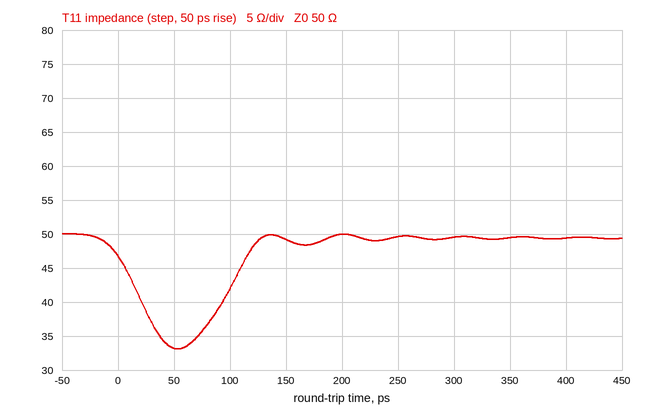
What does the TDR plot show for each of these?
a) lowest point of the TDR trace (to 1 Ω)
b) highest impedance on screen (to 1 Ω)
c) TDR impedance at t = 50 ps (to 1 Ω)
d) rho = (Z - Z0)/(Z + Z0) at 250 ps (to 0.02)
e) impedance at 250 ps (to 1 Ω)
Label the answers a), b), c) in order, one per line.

a) 33 Ω
b) 50 Ω
c) 33 Ω
d) 0.00
e) 50 Ω
